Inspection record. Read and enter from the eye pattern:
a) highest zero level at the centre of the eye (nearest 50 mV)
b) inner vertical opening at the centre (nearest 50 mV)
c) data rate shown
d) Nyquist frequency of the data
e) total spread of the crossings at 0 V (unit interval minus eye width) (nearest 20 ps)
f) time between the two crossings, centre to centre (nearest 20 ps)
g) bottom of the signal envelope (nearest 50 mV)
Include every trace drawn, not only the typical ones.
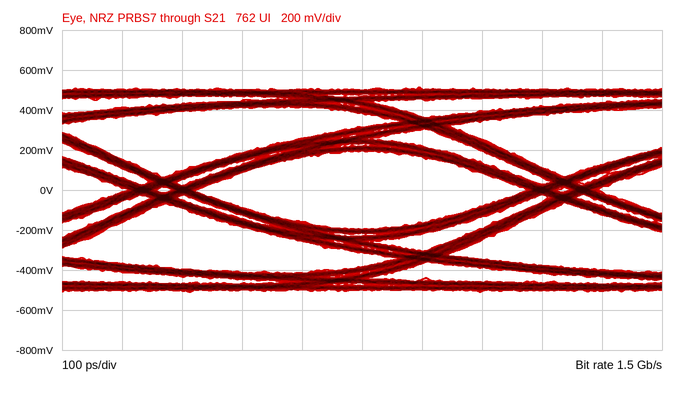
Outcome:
-200 mV
400 mV
1.5 Gb/s
750 MHz
120 ps
660 ps
-500 mV
